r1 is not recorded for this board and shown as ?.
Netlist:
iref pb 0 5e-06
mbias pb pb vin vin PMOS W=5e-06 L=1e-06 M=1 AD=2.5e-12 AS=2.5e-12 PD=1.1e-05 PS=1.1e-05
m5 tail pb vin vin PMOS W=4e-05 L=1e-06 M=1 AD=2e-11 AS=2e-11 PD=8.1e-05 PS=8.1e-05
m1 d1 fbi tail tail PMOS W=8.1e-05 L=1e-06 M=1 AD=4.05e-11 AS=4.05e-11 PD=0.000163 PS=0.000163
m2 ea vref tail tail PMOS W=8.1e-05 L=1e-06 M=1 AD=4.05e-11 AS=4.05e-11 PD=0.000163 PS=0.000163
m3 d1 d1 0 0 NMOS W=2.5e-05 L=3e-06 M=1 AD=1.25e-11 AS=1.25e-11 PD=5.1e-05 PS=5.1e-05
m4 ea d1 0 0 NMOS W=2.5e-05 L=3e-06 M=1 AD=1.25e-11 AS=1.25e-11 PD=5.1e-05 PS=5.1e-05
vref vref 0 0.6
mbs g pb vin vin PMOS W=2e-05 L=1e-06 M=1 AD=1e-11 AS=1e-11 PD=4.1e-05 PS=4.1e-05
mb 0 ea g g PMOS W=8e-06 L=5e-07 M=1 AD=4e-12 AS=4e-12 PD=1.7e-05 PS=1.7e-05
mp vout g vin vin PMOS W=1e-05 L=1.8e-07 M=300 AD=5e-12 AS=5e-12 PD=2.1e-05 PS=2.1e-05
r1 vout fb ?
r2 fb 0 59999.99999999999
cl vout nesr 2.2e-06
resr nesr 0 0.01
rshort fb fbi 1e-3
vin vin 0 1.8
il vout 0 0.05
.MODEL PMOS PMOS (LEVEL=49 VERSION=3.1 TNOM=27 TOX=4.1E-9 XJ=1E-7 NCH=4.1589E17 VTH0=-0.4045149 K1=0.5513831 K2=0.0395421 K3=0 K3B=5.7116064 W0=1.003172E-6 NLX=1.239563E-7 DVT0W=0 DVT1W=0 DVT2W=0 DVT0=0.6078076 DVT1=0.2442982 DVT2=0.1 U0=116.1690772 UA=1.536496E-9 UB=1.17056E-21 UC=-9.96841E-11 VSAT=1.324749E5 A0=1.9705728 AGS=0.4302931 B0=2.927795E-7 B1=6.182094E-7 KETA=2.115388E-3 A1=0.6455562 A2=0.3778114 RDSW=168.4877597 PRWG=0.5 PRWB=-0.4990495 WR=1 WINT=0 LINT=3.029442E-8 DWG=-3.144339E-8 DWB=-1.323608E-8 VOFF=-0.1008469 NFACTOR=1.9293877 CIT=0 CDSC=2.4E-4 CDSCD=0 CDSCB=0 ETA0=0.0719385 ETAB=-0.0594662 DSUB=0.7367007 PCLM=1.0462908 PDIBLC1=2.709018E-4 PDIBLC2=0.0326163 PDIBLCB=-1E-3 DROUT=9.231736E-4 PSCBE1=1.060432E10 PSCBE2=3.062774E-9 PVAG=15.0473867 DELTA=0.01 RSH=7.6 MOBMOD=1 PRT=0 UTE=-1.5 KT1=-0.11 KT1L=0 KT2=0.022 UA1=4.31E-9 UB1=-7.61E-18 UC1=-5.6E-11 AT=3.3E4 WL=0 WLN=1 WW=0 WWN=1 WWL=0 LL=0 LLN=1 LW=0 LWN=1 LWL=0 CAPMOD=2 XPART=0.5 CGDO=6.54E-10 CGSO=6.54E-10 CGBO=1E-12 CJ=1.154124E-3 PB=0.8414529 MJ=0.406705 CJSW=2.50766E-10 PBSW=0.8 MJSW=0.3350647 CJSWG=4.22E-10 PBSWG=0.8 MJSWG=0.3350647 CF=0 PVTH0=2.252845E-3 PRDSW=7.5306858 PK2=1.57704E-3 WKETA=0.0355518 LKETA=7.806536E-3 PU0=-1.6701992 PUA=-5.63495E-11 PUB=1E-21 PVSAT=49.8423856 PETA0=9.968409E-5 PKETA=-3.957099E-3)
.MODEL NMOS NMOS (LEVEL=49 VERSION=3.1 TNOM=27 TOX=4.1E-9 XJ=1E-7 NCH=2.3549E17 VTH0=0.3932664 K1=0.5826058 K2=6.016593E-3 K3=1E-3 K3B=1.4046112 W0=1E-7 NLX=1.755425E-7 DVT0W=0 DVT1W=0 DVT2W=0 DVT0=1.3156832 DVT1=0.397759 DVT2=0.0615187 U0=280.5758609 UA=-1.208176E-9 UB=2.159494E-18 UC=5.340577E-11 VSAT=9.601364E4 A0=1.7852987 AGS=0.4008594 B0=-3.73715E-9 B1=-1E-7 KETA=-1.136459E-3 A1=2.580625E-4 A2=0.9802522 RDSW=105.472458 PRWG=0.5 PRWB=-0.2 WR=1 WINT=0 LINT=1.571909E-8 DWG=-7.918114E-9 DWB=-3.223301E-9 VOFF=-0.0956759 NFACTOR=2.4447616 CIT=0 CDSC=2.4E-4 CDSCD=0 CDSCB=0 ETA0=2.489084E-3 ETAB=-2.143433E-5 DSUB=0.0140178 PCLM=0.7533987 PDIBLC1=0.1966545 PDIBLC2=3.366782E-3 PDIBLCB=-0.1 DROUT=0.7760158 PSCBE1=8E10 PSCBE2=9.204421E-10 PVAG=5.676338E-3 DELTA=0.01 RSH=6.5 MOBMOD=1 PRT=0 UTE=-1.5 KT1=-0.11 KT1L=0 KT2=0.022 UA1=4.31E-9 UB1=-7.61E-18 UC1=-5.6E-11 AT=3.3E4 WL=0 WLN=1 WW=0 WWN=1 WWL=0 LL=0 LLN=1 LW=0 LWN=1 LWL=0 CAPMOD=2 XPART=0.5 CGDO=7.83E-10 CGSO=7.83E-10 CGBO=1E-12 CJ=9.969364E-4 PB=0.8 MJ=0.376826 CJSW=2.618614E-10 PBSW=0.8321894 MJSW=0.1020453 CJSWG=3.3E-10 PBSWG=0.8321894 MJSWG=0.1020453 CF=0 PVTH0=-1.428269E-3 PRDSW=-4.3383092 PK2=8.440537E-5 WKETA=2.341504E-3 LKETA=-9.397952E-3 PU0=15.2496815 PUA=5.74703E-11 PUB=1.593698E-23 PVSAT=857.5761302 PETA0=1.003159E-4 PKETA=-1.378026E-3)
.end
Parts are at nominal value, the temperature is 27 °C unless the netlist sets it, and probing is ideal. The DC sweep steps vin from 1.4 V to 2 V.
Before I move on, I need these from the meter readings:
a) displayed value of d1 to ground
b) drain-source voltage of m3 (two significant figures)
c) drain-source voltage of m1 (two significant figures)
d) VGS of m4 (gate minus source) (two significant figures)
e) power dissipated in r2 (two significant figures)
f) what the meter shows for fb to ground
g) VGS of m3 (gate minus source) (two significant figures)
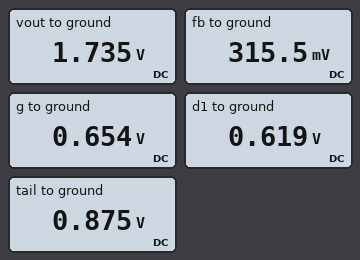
0.619 V
620 mV
-260 mV
620 mV
1.7 µW
315.5 mV
620 mV
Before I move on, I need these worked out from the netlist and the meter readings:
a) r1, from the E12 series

270 kΩ
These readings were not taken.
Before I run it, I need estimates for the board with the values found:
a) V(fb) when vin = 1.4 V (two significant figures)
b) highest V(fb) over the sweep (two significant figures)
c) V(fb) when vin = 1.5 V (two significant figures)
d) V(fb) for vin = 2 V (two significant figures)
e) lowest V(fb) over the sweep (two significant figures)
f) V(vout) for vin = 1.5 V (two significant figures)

64 mV
350 mV
250 mV
350 mV
64 mV
1.4 V
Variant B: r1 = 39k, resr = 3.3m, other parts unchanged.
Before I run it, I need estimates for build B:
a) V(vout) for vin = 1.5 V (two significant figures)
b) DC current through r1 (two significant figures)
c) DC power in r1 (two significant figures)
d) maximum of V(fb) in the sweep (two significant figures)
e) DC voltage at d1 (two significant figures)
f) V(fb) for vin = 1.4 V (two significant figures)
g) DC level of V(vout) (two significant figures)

960 mV
10 µA
3.9 µW
600 mV
560 mV
210 mV
990 mV
